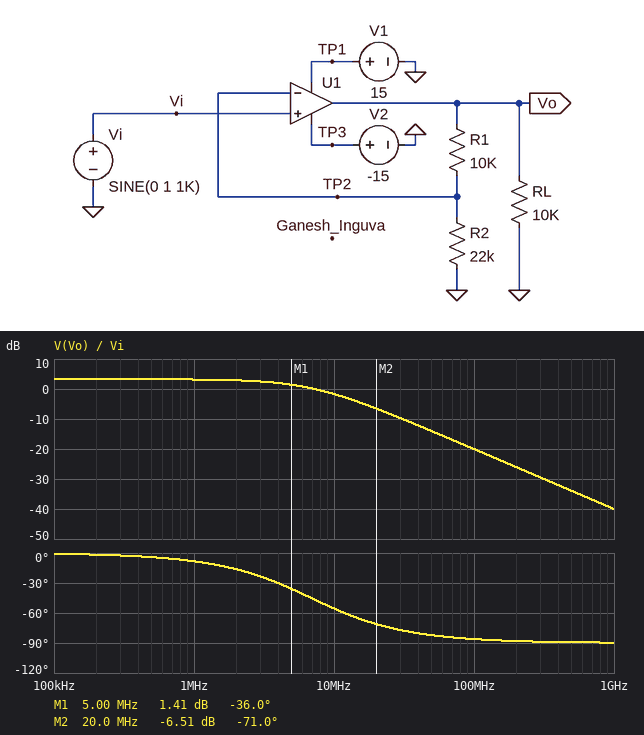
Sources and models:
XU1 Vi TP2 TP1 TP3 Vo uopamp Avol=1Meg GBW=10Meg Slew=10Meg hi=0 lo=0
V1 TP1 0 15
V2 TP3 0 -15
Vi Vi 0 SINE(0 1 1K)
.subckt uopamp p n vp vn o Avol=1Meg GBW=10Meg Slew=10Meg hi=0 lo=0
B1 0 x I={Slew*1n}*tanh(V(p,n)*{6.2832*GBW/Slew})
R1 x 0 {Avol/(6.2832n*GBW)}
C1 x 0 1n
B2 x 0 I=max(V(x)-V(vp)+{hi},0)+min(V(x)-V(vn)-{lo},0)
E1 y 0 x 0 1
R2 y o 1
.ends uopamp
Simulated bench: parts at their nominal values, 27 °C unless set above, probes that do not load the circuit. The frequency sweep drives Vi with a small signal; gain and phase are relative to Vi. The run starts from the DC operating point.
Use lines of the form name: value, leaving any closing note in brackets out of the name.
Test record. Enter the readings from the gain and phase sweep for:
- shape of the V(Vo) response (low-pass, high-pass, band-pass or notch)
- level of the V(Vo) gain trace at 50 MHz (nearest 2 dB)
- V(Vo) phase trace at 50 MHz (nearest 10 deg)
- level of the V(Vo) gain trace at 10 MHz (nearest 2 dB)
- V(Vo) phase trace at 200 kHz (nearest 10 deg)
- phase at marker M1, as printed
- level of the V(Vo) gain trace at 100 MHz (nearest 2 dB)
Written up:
shape of the V(Vo) response: low-pass
level of the V(Vo) gain trace at 50 MHz: -14 dB
V(Vo) phase trace at 50 MHz: -80 deg
level of the V(Vo) gain trace at 10 MHz: -2 dB
V(Vo) phase trace at 200 kHz: 0 deg
phase at marker M1, as printed: -36.0 deg
level of the V(Vo) gain trace at 100 MHz: -20 dB
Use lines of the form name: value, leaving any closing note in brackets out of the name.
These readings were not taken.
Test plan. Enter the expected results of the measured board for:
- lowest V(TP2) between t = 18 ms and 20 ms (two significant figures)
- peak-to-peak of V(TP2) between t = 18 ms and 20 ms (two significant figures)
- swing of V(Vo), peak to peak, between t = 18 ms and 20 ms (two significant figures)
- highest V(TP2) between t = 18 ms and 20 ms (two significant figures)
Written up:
lowest V(TP2) between t = 18 ms and 20 ms: -1.0 V
peak-to-peak of V(TP2) between t = 18 ms and 20 ms: 2.0 V
swing of V(Vo), peak to peak, between t = 18 ms and 20 ms: 2.9 V
highest V(TP2) between t = 18 ms and 20 ms: 1.0 V
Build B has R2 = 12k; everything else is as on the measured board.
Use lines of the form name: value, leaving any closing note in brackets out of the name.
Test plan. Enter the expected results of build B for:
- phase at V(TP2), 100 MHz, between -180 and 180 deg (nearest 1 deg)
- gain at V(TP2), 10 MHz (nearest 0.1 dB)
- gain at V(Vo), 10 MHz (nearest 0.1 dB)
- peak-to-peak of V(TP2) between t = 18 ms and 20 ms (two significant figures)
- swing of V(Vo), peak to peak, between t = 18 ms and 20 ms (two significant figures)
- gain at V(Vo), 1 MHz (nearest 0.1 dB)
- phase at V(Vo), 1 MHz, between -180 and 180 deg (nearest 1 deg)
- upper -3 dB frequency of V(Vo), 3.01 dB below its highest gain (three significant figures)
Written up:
phase at V(TP2), 100 MHz, between -180 and 180 deg: -87 deg
gain at V(TP2), 10 MHz: -6.4 dB
gain at V(Vo), 10 MHz: -1.1 dB
peak-to-peak of V(TP2) between t = 18 ms and 20 ms: 2.0 V
swing of V(Vo), peak to peak, between t = 18 ms and 20 ms: 3.7 V
gain at V(Vo), 1 MHz: 5.1 dB
phase at V(Vo), 1 MHz, between -180 and 180 deg: -10 deg
upper -3 dB frequency of V(Vo), 3.01 dB below its highest gain: 5.45 MHz
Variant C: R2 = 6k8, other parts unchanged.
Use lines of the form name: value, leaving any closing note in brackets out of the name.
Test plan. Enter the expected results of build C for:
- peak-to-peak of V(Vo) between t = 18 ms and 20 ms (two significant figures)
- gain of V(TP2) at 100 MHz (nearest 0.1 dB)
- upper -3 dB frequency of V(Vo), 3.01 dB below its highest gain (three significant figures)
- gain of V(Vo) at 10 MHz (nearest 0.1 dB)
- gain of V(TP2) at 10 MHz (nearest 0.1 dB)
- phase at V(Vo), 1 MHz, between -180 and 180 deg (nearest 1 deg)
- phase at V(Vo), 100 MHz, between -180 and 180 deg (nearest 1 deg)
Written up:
peak-to-peak of V(Vo) between t = 18 ms and 20 ms: 4.9 V
gain of V(TP2) at 100 MHz: -27.9 dB
upper -3 dB frequency of V(Vo), 3.01 dB below its highest gain: 4.05 MHz
gain of V(Vo) at 10 MHz: -0.7 dB
gain of V(TP2) at 10 MHz: -8.5 dB
phase at V(Vo), 1 MHz, between -180 and 180 deg: -14 deg
phase at V(Vo), 100 MHz, between -180 and 180 deg: -88 deg
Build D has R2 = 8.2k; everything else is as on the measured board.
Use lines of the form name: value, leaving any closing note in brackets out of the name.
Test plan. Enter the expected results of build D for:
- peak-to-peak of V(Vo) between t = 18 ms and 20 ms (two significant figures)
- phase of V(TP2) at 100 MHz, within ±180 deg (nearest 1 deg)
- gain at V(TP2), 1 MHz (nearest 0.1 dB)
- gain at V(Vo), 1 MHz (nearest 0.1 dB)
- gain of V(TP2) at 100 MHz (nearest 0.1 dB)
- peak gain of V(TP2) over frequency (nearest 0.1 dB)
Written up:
peak-to-peak of V(Vo) between t = 18 ms and 20 ms: 4.4 V
phase of V(TP2) at 100 MHz, within ±180 deg: -87 deg
gain at V(TP2), 1 MHz: -0.2 dB
gain at V(Vo), 1 MHz: 6.7 dB
gain of V(TP2) at 100 MHz: -26.9 dB
peak gain of V(TP2) over frequency: 0 dB
